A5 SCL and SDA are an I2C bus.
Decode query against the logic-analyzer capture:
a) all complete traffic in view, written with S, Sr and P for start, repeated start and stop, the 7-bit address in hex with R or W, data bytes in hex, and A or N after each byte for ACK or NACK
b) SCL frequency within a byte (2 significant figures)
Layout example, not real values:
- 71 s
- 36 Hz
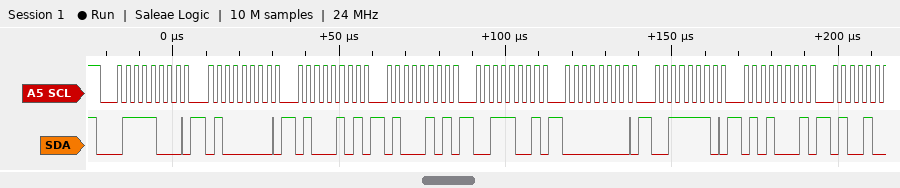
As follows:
- S 3CW A 40 A 45 A 45 A 39 A 00 A 3E A 51 A
- 400 kHz
